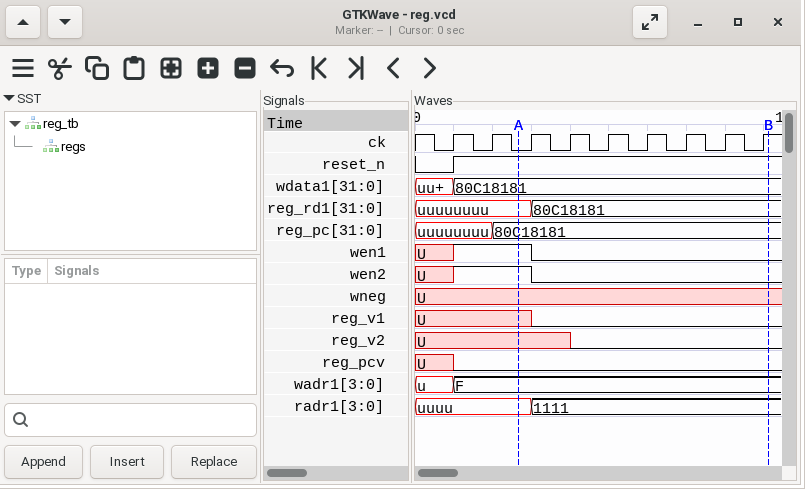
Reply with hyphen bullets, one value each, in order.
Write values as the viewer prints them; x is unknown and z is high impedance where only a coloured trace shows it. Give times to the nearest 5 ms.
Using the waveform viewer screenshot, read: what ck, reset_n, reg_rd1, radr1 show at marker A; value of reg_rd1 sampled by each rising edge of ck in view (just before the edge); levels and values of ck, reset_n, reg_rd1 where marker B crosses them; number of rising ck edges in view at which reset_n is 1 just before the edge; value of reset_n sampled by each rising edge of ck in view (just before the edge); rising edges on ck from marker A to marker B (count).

- ck=0, reset_n=1, reg_rd1=uuuuuuuu, radr1=uuuu
- uuuuuuuu, uuuuuuuu, uuuuuuuu, 80C18181, 80C18181, 80C18181, 80C18181, 80C18181, 80C18181
- ck=1, reset_n=1, reg_rd1=80C18181
- 8
- 0 1 1 1 1 1 1 1 1
- 7
